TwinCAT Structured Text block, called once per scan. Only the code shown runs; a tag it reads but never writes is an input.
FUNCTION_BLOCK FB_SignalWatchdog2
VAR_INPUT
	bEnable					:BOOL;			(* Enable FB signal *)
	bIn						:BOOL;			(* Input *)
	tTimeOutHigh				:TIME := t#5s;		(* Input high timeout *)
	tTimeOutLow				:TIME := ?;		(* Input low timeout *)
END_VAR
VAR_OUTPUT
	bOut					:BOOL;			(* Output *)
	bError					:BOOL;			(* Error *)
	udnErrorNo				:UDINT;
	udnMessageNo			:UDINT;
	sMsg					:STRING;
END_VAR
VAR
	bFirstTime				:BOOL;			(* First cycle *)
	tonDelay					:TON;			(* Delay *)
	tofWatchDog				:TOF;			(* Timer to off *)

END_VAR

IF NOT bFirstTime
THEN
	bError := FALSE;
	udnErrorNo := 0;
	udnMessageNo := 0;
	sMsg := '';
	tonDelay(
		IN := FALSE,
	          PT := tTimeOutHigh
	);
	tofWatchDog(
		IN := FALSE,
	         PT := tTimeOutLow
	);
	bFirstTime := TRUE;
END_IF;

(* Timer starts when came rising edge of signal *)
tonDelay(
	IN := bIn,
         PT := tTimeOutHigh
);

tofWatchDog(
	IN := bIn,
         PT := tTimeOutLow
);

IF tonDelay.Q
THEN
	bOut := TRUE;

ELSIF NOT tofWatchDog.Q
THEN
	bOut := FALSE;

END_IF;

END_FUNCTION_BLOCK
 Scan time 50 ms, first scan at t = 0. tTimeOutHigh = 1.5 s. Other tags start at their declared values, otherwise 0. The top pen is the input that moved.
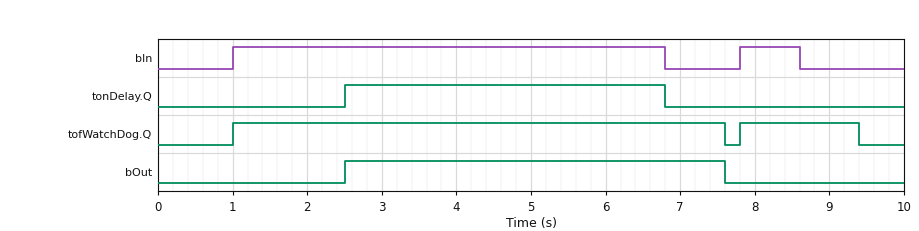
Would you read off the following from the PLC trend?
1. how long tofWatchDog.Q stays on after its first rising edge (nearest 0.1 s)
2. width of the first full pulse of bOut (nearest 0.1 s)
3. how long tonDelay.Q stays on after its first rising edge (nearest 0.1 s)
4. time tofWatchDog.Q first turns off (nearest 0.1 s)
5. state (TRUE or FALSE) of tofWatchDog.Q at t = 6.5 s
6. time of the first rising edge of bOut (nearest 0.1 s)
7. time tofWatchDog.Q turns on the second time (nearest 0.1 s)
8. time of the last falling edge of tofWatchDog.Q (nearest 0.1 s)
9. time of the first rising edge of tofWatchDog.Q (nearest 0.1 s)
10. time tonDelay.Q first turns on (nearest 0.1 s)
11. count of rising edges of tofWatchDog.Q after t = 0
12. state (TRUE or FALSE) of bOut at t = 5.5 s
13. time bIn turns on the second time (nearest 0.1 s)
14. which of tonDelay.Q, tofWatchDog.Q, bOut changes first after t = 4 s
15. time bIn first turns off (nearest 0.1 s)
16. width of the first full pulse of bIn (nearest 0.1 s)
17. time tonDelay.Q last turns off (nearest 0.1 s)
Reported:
6.6 s
5.1 s
4.3 s
7.6 s
TRUE
2.5 s
7.8 s
9.4 s
1.0 s
2.5 s
2
TRUE
7.8 s
tonDelay.Q
6.8 s
5.8 s
6.8 s
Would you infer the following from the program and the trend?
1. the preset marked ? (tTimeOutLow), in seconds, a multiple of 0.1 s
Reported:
0.8 s
